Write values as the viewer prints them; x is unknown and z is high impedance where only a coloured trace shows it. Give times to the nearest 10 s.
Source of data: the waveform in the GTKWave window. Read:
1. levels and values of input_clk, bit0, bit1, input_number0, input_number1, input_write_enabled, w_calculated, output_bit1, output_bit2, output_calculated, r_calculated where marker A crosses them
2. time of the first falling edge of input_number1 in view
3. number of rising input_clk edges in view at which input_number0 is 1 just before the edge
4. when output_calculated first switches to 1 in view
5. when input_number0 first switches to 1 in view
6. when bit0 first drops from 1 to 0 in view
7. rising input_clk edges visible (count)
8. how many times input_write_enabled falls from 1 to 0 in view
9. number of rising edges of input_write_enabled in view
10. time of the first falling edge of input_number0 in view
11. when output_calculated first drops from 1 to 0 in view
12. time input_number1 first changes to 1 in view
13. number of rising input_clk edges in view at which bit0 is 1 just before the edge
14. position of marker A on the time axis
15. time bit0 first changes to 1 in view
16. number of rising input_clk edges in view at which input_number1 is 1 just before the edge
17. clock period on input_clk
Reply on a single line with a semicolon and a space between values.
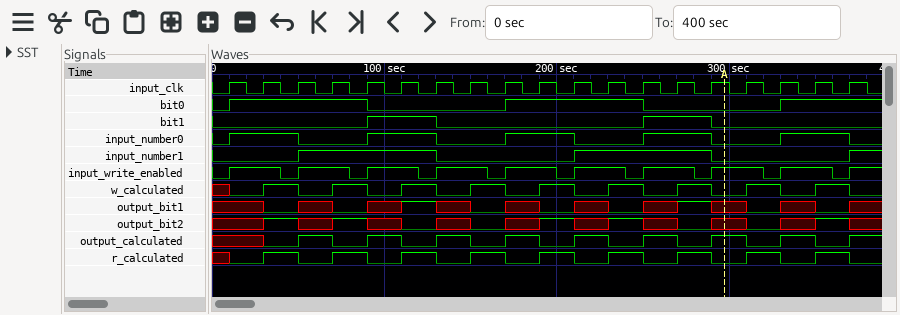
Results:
input_clk=1, bit0=0, bit1=0, input_number0=0, input_number1=0, input_write_enabled=1, w_calculated=0, output_bit1=x, output_bit2=x, output_calculated=1, r_calculated=0; 130 s; 10; 50 s; 10 s; 90 s; 19; 9; 10; 50 s; 70 s; 50 s; 10; 300 s; 10 s; 8; 20 s
